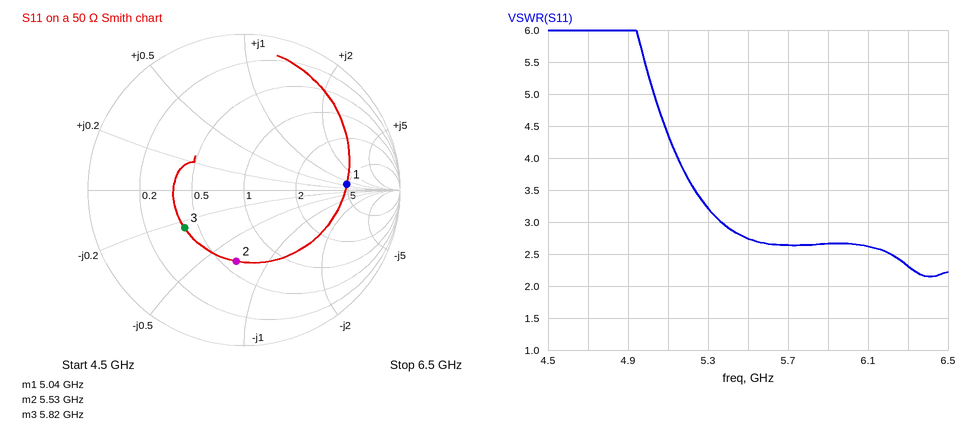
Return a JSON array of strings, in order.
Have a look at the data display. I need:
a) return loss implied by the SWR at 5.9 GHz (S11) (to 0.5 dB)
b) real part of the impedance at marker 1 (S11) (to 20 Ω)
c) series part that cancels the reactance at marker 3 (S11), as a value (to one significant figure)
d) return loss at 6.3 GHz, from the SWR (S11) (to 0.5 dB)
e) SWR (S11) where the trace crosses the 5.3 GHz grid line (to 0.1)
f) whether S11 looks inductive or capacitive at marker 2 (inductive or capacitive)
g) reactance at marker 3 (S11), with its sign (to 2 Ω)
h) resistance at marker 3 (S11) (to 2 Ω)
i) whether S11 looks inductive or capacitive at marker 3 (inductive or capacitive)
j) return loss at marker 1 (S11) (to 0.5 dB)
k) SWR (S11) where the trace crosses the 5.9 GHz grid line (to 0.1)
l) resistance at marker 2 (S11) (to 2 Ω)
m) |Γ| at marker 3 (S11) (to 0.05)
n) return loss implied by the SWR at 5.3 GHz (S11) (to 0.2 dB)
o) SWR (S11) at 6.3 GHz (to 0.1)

["7.0 dB", "240 Ω", "300 pH", "8.0 dB", "3.2", "capacitive", "-12 Ω", "20 Ω", "capacitive", "3.5 dB", "2.7", "30 Ω", "0.45", "5.6 dB", "2.3"]
